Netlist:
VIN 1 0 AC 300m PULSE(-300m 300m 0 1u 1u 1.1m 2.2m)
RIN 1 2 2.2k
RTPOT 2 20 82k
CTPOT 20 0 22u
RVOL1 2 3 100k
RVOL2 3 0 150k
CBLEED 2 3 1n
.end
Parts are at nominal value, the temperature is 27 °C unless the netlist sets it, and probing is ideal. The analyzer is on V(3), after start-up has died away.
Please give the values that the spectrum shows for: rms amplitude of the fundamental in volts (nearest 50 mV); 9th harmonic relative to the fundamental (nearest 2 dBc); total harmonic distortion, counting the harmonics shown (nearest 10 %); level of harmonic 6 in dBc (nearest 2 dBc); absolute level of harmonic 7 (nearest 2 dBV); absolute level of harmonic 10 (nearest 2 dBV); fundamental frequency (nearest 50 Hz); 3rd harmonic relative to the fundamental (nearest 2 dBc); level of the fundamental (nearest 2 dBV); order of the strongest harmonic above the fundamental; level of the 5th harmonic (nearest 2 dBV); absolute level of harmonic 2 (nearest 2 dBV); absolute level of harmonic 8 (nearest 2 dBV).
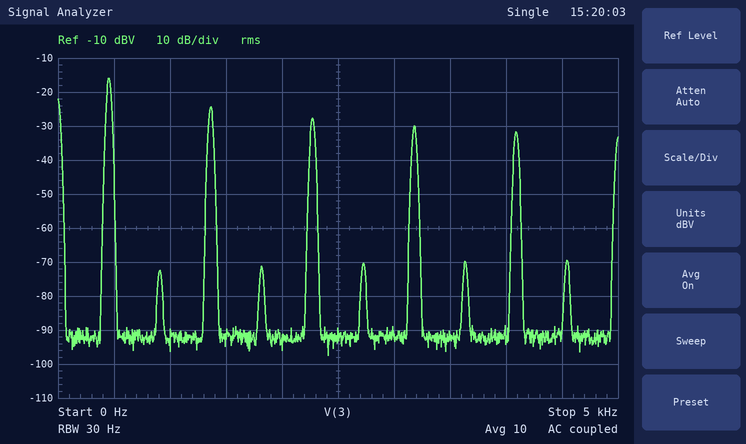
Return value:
150 mV
-16 dBc
50 %
-54 dBc
-30 dBV
-70 dBV
450 Hz
-8 dBc
-16 dBV
3
-28 dBV
-72 dBV
-70 dBV
